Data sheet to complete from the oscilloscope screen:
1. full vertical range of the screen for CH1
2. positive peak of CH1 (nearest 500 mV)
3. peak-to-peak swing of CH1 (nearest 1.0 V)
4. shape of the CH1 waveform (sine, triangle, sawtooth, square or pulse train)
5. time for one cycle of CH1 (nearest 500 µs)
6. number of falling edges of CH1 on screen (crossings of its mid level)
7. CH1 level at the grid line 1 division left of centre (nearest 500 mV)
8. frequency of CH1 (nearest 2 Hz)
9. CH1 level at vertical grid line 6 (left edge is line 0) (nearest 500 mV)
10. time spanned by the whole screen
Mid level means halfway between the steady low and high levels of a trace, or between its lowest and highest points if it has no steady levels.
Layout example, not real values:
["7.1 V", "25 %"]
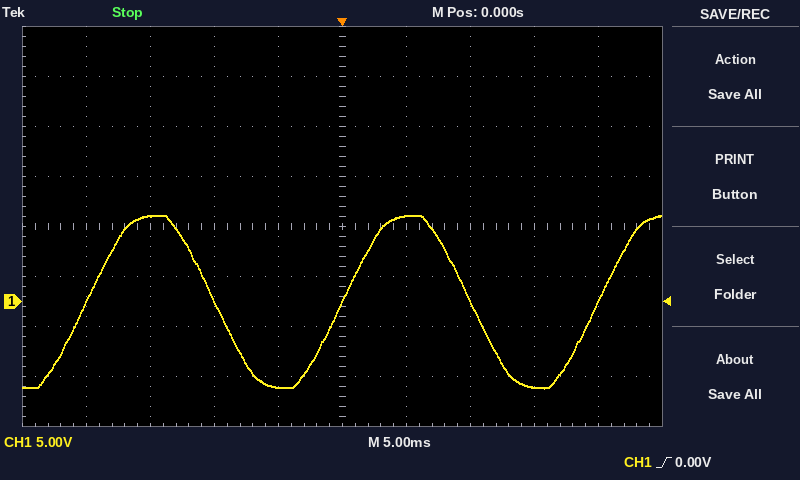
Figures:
["40 V", "8.5 V", "17.0 V", "sine", "20.0 ms", "2", "-8.5 V", "50 Hz", "8.5 V", "50 ms"]
